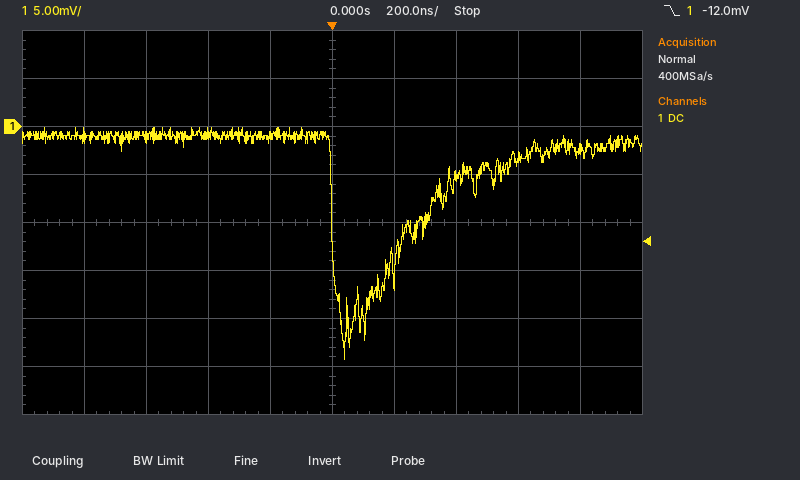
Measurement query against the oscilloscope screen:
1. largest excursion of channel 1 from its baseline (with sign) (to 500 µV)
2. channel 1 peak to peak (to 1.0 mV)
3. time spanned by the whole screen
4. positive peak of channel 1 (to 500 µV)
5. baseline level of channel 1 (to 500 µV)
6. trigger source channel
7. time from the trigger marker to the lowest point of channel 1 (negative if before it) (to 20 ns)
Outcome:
-23.0 mV
24.0 mV
2 µs
0.0 mV
-1.0 mV
channel 1
+40 ns
